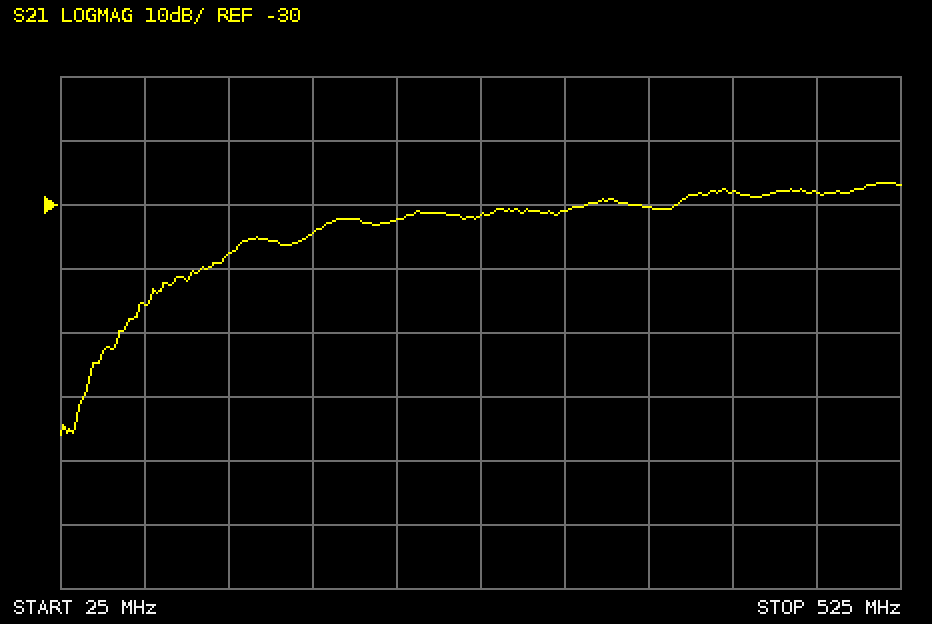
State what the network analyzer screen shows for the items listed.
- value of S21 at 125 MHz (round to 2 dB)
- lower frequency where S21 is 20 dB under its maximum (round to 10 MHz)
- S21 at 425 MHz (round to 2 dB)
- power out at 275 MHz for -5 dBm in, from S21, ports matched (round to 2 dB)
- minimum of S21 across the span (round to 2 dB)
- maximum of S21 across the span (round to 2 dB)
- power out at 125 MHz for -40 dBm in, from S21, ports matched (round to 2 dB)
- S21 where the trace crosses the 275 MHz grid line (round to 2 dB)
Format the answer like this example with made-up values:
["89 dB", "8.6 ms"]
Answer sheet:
["-38 dB", "70 MHz", "-28 dB", "-36 dBm", "-66 dB", "-26 dB", "-78 dBm", "-32 dB"]
